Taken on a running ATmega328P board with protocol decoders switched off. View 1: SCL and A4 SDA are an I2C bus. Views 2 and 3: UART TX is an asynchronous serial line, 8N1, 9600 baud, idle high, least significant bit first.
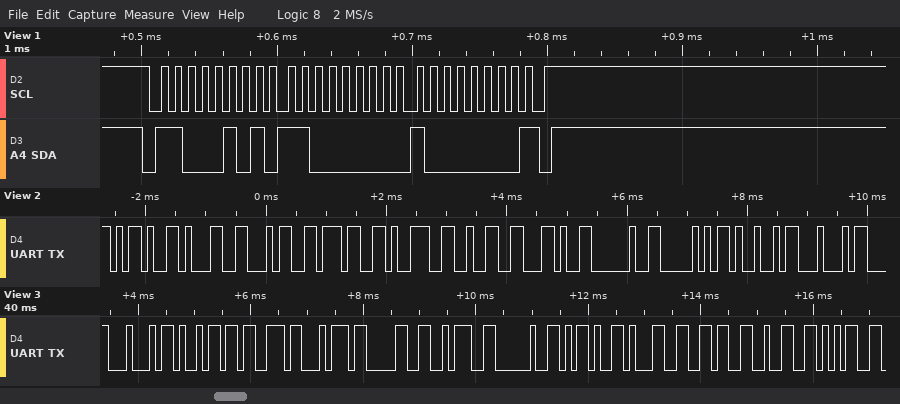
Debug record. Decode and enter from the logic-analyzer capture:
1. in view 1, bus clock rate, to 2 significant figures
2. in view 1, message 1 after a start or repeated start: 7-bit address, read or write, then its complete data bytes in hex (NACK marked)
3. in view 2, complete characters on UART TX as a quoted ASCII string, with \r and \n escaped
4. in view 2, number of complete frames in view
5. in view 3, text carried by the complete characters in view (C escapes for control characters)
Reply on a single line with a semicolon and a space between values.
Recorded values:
100 kHz; 0x62 read: C0 80 NACK; "-14792, PID"; 11; "Dist0: -1625"
